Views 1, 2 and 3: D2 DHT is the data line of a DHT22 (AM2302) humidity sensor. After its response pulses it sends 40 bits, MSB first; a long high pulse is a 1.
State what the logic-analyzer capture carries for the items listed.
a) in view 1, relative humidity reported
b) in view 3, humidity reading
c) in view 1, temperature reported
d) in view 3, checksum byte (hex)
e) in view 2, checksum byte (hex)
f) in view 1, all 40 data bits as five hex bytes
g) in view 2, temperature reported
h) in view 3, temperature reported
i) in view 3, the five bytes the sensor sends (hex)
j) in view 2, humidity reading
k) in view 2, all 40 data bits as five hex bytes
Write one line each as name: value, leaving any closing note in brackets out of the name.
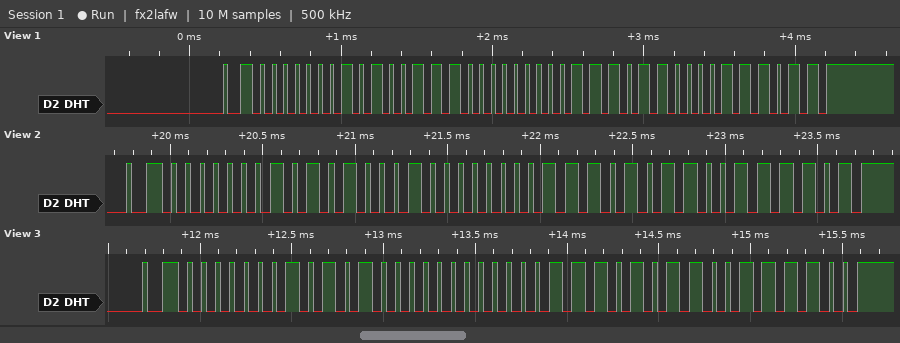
in view 1, relative humidity reported: 33.4 %
in view 3, humidity reading: 33.6 %
in view 1, temperature reported: 23.6 °C
in view 3, checksum byte: 0x3C
in view 2, checksum byte: 0x3D
in view 1, all 40 data bits as five hex bytes: 01 4E 00 EC 3B
in view 2, temperature reported: 23.5 °C
in view 3, temperature reported: 23.5 °C
in view 3, the five bytes the sensor sends: 01 50 00 EB 3C
in view 2, humidity reading: 33.7 %
in view 2, all 40 data bits as five hex bytes: 01 51 00 EB 3D
